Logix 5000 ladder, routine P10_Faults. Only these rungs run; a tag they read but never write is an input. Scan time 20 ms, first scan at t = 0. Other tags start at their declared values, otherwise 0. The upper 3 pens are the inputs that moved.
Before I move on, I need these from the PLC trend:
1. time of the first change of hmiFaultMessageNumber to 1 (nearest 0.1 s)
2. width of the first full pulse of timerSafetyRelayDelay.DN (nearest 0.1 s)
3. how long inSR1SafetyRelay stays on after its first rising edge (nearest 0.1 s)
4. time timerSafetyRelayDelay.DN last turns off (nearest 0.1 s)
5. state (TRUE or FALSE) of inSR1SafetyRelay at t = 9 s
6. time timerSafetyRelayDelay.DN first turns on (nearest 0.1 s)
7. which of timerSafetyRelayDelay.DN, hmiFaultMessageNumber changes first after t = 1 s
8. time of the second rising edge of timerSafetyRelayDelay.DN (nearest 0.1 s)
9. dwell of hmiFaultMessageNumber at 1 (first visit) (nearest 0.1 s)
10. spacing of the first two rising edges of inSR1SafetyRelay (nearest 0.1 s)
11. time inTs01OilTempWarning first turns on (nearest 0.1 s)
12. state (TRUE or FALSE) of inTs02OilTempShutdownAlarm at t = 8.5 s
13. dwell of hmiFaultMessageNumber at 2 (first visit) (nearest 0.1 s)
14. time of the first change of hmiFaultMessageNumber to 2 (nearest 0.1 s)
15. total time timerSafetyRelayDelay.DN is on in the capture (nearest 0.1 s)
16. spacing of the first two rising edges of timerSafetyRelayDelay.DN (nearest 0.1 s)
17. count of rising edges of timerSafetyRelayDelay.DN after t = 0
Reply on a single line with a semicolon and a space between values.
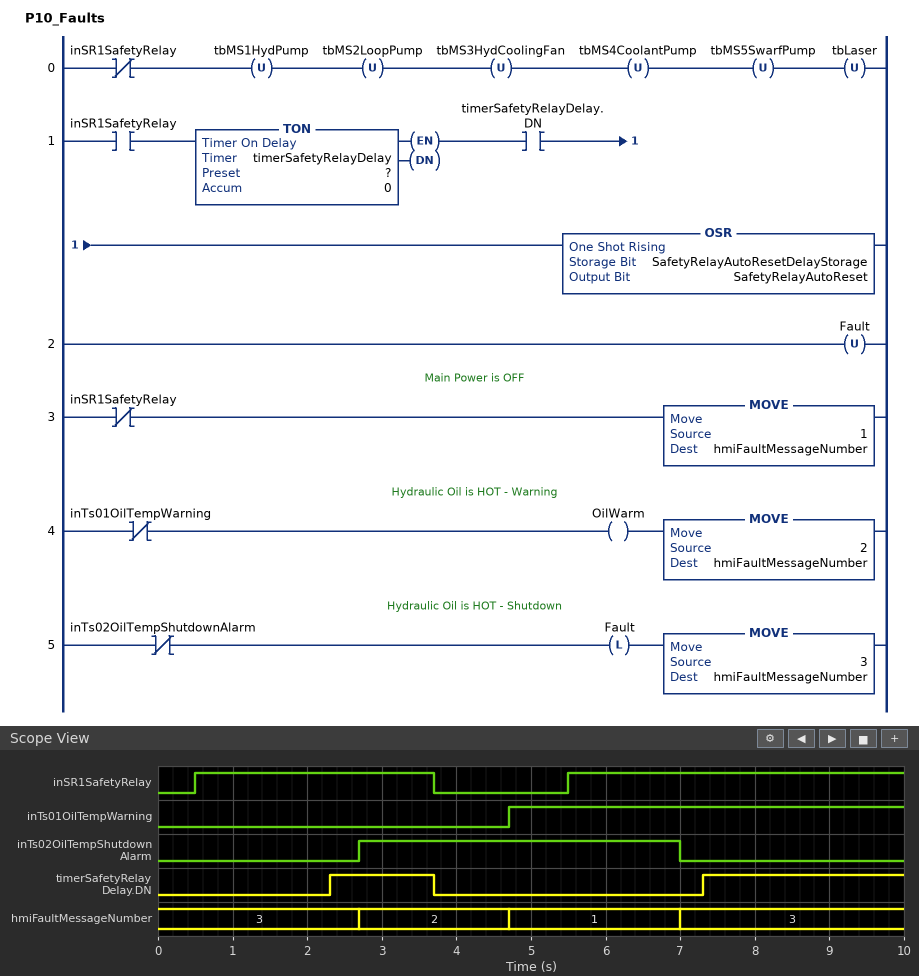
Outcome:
4.7 s; 1.4 s; 3.2 s; 3.7 s; TRUE; 2.3 s; timerSafetyRelayDelay.DN; 7.3 s; 2.3 s; 5.0 s; 4.7 s; FALSE; 2.0 s; 2.7 s; 4.1 s; 5.0 s; 2
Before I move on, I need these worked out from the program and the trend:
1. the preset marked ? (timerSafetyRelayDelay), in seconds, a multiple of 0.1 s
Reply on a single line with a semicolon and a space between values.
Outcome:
1.8 s
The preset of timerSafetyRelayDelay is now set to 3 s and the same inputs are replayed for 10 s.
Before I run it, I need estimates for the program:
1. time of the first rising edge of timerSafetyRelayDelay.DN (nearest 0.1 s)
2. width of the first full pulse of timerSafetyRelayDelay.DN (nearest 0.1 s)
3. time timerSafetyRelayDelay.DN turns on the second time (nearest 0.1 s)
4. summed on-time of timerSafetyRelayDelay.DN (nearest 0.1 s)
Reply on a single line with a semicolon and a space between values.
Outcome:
3.5 s; 0.2 s; 8.5 s; 1.7 s
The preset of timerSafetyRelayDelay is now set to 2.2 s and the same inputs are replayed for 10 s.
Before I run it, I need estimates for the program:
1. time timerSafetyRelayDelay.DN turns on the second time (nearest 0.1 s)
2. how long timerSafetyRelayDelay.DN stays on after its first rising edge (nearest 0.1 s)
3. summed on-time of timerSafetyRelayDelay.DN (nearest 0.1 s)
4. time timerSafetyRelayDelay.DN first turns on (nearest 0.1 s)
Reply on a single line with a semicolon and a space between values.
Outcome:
7.7 s; 1.0 s; 3.3 s; 2.7 s
